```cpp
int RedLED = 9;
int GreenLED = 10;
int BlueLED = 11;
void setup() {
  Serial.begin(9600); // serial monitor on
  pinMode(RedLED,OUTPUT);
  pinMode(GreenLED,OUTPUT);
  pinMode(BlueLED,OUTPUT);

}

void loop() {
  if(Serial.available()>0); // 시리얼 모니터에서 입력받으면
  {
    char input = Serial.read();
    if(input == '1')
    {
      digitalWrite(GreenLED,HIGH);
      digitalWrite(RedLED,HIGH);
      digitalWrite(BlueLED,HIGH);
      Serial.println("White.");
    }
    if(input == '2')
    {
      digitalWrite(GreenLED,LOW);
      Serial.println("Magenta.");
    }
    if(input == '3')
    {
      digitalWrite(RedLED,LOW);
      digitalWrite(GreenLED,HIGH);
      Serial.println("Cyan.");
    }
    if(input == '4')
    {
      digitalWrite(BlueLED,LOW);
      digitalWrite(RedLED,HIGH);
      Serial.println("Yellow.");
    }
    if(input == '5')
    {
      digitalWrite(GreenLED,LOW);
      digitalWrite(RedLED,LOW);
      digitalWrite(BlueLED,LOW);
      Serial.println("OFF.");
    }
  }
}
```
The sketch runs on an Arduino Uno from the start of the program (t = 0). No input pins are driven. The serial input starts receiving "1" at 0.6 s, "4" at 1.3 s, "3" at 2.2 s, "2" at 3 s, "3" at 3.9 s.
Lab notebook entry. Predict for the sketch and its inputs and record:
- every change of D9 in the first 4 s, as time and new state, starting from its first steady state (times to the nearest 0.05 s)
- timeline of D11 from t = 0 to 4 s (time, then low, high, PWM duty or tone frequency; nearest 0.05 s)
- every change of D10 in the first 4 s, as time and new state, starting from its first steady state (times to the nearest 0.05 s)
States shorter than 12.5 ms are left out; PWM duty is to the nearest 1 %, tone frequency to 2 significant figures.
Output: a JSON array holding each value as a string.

["0 s low; 0.6 s high; 2.2 s low", "0 s low; 0.6 s high; 1.3 s low", "0 s low; 0.6 s high; 3 s low; 3.9 s high"]
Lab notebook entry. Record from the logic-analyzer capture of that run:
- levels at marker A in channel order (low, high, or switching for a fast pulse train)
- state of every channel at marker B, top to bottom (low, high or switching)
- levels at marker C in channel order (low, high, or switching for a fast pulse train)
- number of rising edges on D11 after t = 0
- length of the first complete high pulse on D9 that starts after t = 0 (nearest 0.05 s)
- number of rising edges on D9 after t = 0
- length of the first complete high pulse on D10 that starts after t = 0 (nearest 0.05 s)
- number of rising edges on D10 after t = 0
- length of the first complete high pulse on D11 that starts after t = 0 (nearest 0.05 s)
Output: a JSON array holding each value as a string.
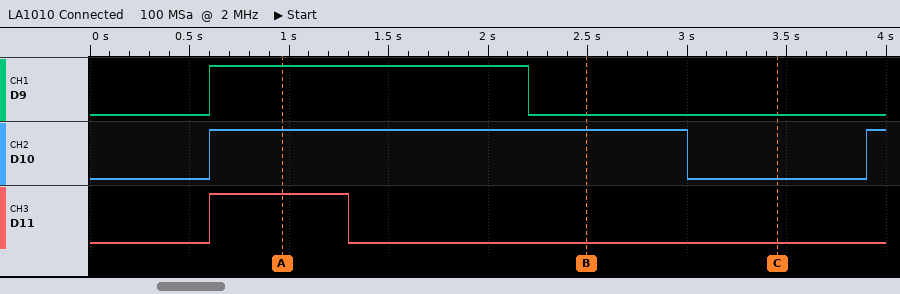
["D9 high, D10 high, D11 high", "D9 low, D10 high, D11 low", "D9 low, D10 low, D11 low", "1", "1.60 s", "1", "2.40 s", "2", "0.70 s"]
